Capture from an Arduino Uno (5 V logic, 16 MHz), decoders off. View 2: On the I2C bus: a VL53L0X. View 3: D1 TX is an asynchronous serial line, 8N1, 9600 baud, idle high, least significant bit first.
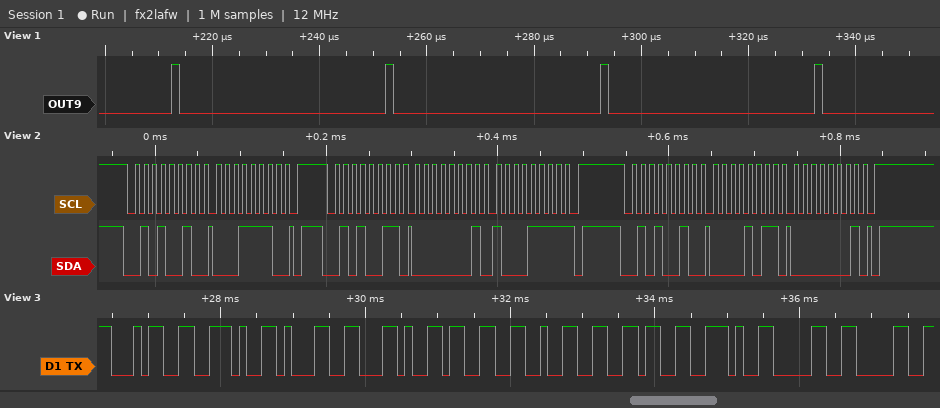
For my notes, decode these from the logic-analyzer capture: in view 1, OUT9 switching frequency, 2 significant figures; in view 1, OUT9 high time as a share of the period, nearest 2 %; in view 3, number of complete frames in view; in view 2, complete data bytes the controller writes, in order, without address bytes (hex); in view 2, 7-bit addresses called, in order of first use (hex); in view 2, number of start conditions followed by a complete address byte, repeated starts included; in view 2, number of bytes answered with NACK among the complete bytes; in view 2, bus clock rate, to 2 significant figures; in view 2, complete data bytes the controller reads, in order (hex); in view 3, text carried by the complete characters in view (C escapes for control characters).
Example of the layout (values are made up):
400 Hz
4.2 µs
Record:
25 kHz
4 %
10
1E 0B 01
0x29
3
1
100 kHz
01 8F
"4.1,326.00"
